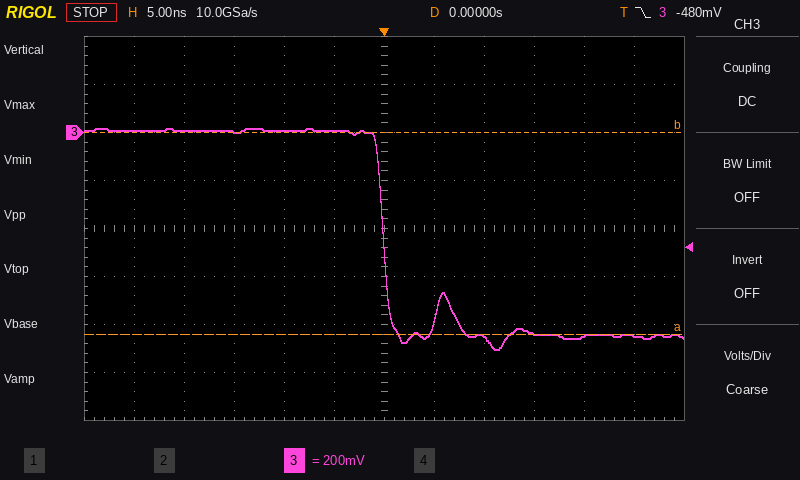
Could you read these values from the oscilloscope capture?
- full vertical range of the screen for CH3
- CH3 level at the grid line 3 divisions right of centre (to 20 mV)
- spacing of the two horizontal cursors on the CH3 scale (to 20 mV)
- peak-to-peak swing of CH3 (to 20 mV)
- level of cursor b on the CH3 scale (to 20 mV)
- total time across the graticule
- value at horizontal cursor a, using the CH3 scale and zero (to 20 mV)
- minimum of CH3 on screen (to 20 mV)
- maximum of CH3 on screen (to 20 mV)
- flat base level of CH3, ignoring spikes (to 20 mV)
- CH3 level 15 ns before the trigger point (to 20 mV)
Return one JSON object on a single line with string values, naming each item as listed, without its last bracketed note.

{"full vertical range of the screen for CH3": "1.6 V", "CH3 level at the grid line 3 divisions right of centre": "-840 mV", "spacing of the two horizontal cursors on the CH3 scale": "840 mV", "peak-to-peak swing of CH3": "920 mV", "level of cursor b on the CH3 scale": "0 mV", "total time across the graticule": "60 ns", "value at horizontal cursor a, using the CH3 scale and zero": "-840 mV", "minimum of CH3 on screen": "-900 mV", "maximum of CH3 on screen": "20 mV", "flat base level of CH3, ignoring spikes": "-840 mV", "CH3 level 15 ns before the trigger point": "0 mV"}
